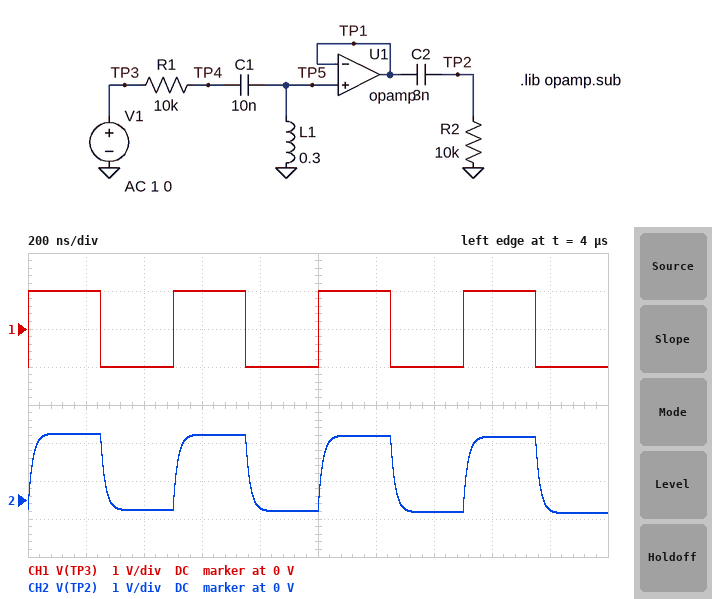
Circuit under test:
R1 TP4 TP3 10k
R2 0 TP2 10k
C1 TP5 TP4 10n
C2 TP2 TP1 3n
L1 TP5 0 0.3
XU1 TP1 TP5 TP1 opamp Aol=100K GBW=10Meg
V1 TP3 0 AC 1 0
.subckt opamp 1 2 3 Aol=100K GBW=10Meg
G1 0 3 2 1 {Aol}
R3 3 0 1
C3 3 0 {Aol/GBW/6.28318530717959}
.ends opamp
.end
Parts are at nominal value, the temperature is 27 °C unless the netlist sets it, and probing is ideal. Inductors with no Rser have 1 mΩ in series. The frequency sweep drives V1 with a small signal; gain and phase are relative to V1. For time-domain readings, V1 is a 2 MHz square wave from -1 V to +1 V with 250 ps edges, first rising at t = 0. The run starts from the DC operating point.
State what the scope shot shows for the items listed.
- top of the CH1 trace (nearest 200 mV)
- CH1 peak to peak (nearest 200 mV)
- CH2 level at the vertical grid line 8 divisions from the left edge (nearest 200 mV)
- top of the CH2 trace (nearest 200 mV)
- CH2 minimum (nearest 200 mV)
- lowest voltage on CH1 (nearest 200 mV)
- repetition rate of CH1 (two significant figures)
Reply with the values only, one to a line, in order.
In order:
1.0 V
2.0 V
1.6 V
1.8 V
-400 mV
-1.0 V
2.0 MHz
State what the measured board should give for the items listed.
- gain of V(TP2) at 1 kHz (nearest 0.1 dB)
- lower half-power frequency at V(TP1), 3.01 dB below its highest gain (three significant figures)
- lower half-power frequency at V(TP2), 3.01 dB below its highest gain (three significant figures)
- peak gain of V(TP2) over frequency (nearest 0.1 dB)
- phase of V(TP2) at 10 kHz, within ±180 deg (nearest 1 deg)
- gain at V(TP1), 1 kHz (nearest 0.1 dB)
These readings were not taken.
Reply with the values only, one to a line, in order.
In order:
-33.9 dB
3.97 kHz
6.94 kHz
0 dB
58 deg
-19.2 dB
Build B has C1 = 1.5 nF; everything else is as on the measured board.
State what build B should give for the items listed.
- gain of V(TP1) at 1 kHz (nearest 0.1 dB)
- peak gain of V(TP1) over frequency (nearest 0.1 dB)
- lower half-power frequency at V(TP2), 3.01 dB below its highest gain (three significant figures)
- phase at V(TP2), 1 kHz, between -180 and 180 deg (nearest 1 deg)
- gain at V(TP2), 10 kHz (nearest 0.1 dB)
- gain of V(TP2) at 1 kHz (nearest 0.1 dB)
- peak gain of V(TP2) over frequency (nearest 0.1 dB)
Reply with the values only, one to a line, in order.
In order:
-34.9 dB
3.6 dB
6.62 kHz
-106 deg
2.2 dB
-49.5 dB
2.3 dB
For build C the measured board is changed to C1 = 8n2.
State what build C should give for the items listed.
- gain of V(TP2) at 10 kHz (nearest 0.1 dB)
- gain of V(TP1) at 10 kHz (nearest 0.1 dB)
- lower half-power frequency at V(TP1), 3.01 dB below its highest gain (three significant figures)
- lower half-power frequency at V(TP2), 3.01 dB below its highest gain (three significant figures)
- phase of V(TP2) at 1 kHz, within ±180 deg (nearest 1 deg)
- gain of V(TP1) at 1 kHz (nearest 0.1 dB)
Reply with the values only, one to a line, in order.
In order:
-1.4 dB
-0.4 dB
3.84 kHz
6.66 kHz
-130 deg
-20.6 dB
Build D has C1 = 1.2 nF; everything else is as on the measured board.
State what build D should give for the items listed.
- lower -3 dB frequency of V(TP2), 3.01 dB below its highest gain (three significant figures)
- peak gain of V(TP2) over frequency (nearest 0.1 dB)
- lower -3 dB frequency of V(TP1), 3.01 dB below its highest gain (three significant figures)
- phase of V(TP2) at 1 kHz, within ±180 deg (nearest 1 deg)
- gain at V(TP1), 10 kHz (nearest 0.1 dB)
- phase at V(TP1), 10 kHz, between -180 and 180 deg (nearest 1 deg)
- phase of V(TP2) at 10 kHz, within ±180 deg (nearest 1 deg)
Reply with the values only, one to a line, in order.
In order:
7.33 kHz
3.3 dB
7.09 kHz
-105 deg
4.3 dB
61 deg
89 deg
